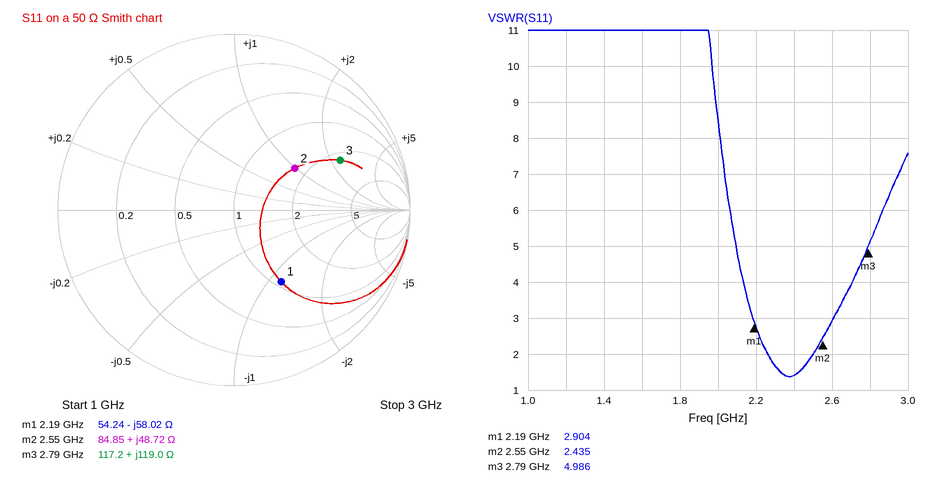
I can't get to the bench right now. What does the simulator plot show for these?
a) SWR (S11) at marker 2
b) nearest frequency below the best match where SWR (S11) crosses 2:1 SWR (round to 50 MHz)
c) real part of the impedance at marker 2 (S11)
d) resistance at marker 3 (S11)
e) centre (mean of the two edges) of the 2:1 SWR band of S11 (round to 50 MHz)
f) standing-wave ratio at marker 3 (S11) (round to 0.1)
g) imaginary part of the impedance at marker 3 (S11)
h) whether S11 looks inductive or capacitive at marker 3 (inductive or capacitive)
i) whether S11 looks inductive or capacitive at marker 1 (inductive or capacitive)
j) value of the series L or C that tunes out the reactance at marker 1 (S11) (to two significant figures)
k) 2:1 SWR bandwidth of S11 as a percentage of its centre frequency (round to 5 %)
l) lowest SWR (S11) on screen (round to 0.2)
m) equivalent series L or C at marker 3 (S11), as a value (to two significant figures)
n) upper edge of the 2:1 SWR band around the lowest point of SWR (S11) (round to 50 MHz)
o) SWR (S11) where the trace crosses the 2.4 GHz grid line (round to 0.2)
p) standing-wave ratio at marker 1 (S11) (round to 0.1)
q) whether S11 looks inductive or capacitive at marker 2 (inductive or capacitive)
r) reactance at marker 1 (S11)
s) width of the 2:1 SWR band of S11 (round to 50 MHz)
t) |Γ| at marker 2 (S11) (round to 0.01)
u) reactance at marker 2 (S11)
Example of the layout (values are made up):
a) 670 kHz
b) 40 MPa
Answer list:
a) 2.435
b) 2.25 GHz
c) 84.85 Ω
d) 117.2 Ω
e) 2.40 GHz
f) 5.0
g) +119.0 Ω
h) inductive
i) capacitive
j) 4.2 nH
k) 10 %
l) 1.4
m) 6.8 nH
n) 2.50 GHz
o) 1.4
p) 2.9
q) inductive
r) -58.02 Ω
s) 250 MHz
t) 0.42
u) +48.72 Ω
